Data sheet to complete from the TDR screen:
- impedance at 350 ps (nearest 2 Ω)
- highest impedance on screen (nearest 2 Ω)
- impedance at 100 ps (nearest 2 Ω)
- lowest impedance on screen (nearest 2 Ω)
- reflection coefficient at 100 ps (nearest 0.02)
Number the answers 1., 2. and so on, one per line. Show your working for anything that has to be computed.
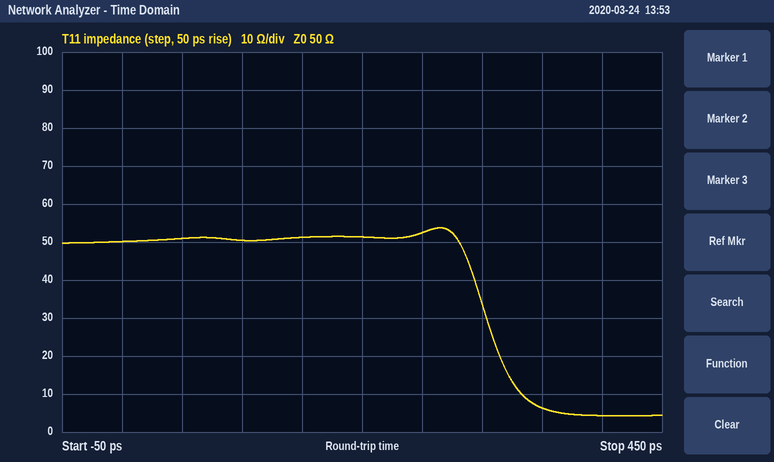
1. 6 Ω
2. 54 Ω
3. 50 Ω
4. 4 Ω
5. (50 − 50)/(50 + 50) ≈ 0.00
